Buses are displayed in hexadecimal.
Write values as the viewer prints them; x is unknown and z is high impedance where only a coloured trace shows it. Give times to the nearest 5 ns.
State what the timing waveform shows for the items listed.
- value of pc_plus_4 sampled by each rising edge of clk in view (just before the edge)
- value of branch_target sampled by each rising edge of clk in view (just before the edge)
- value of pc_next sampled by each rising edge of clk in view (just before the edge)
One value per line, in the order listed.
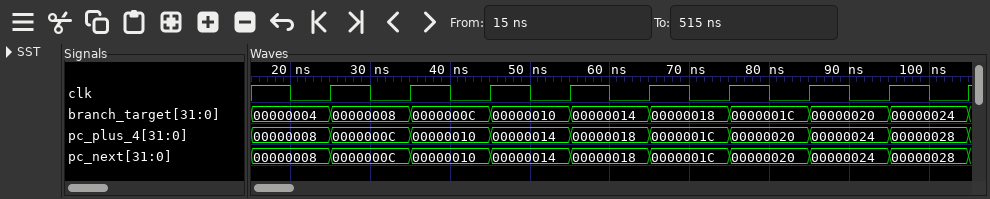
00000008, 0000000C, 00000010, 00000014, 00000018, 0000001C, 00000020, 00000024, 00000028
00000004, 00000008, 0000000C, 00000010, 00000014, 00000018, 0000001C, 00000020, 00000024
00000008, 0000000C, 00000010, 00000014, 00000018, 0000001C, 00000020, 00000024, 00000028
